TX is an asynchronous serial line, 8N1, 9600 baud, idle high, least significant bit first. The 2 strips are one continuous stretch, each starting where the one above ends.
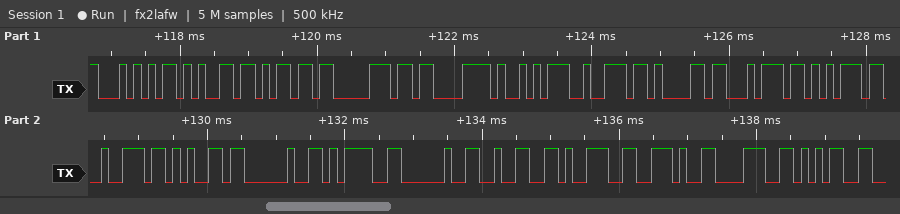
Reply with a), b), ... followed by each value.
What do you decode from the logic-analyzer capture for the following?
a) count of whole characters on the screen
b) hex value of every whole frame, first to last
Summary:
a) 20
b) 0x54 0x65 0x6D 0x70 0xC3 0xA9 0x72 0x61 0x74 0x75 0x72 0x65 0x20 0x3D 0x20 0x32 0x39 0x2E 0x38 0x35
